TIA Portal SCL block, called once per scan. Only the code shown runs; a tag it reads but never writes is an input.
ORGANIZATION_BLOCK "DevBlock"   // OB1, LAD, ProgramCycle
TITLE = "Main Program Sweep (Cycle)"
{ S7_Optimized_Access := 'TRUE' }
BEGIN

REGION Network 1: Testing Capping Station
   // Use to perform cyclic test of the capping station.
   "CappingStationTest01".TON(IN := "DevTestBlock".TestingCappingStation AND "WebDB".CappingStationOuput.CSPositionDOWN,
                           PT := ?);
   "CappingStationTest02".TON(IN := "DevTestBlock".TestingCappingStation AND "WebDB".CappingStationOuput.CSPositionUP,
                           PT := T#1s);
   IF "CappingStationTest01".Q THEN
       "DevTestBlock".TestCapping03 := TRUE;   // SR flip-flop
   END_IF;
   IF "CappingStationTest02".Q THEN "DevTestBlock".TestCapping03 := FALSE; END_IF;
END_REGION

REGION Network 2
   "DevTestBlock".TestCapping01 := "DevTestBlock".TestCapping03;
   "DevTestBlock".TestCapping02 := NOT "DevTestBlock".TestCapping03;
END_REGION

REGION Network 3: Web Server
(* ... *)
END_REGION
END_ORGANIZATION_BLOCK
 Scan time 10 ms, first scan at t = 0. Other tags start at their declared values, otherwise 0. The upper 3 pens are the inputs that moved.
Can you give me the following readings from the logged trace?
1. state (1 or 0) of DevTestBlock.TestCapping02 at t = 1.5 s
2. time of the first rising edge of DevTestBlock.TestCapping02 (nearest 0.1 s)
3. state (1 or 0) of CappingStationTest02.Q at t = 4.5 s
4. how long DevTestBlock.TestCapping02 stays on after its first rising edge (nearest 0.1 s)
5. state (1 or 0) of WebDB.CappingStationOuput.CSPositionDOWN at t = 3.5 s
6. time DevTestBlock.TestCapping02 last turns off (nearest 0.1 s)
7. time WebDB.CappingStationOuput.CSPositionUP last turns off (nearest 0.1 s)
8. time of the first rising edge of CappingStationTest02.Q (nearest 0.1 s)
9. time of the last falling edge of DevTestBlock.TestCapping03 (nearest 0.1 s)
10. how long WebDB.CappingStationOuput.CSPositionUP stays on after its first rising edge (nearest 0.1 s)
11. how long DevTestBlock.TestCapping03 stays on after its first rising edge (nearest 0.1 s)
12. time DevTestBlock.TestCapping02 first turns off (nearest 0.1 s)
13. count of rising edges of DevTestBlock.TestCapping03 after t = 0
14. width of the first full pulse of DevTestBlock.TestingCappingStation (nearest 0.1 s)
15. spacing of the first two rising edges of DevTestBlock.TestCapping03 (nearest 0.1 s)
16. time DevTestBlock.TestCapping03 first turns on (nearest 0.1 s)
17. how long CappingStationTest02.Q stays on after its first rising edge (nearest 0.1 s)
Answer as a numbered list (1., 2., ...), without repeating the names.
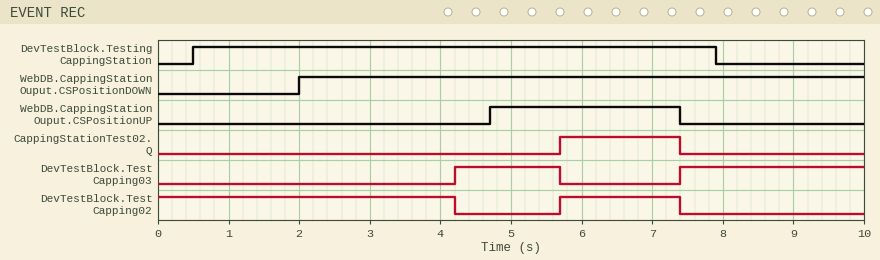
1. 1
2. 5.7 s
3. 0
4. 1.7 s
5. 1
6. 7.4 s
7. 7.4 s
8. 5.7 s
9. 5.7 s
10. 2.7 s
11. 1.5 s
12. 4.2 s
13. 2
14. 7.4 s
15. 3.2 s
16. 4.2 s
17. 1.7 s
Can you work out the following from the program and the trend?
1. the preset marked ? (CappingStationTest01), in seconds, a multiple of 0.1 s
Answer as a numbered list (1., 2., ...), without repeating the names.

1. 2.2 s
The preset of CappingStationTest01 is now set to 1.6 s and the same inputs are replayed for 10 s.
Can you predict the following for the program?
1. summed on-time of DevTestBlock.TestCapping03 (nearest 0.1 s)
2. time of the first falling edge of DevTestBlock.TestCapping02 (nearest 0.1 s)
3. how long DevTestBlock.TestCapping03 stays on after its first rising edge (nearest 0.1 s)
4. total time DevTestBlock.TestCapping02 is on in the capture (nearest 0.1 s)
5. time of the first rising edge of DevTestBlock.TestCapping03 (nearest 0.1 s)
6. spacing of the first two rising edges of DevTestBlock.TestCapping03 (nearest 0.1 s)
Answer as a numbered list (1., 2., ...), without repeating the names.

1. 4.7 s
2. 3.6 s
3. 2.1 s
4. 5.3 s
5. 3.6 s
6. 3.8 s
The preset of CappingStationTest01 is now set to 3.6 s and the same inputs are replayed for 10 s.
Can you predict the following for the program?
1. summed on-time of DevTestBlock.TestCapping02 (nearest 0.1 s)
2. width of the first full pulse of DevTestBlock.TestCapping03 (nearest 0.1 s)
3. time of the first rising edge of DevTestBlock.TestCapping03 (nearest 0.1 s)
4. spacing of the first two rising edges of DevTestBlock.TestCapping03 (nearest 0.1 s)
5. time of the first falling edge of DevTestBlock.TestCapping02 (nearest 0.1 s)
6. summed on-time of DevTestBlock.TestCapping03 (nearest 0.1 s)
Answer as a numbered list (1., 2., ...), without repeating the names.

1. 7.3 s
2. 0.1 s
3. 5.6 s
4. 1.8 s
5. 5.6 s
6. 2.7 s
